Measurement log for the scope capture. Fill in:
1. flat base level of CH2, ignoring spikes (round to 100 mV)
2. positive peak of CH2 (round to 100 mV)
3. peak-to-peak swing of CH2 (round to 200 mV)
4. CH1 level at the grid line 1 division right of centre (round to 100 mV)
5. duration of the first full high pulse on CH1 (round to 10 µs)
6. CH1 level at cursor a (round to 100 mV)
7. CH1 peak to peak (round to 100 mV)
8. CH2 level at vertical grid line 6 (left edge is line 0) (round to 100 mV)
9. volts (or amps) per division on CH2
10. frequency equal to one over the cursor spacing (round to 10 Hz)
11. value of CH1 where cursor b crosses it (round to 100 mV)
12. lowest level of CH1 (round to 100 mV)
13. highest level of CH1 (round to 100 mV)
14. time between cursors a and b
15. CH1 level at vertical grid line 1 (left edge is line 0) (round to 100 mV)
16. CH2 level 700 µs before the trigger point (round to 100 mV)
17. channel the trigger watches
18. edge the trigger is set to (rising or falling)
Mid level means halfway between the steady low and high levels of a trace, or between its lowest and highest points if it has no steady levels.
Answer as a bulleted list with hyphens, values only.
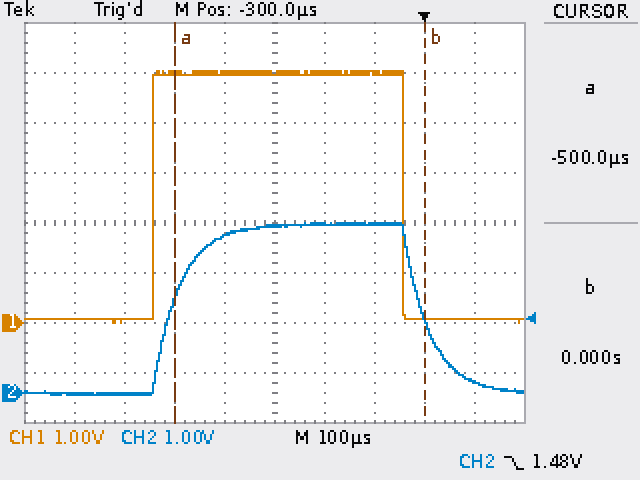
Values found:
- 0.0 V
- 3.4 V
- 3.4 V
- 5.0 V
- 500 µs
- 5.0 V
- 5.0 V
- 3.4 V
- 1 V
- 2.00 kHz
- 100 mV
- 0.0 V
- 5.0 V
- 500 µs
- 100 mV
- 0.0 V
- CH2
- falling
